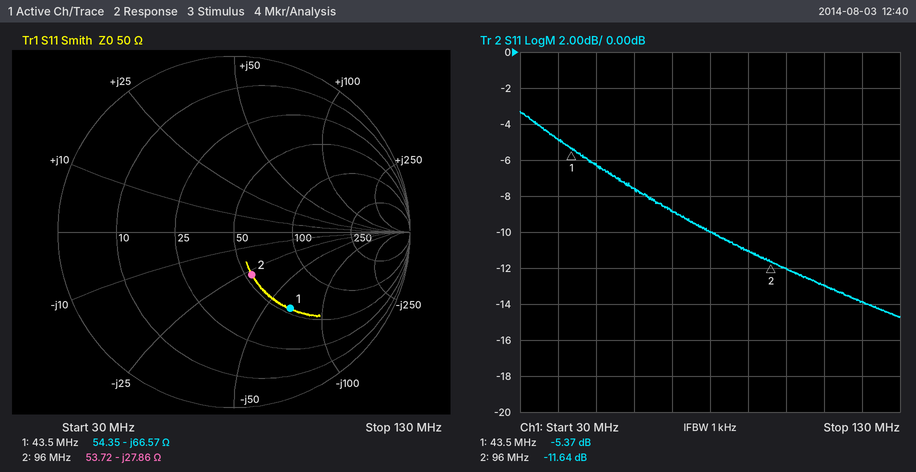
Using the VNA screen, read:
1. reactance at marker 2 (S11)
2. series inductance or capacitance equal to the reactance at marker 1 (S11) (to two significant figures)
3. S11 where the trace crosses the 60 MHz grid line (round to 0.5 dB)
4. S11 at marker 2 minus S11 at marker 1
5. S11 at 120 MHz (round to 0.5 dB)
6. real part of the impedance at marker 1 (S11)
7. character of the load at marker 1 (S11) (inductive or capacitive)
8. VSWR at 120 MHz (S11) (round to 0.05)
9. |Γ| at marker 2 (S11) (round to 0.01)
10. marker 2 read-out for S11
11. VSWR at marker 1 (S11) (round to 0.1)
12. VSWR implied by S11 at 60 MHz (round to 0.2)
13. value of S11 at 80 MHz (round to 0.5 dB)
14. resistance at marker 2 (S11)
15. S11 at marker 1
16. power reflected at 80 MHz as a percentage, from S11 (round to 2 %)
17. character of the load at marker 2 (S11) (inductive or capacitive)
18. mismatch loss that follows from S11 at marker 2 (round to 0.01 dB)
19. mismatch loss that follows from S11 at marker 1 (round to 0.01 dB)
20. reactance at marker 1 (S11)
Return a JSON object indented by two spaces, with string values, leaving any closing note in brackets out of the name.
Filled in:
{
  "reactance at marker 2": "-27.86 Ω",
  "series inductance or capacitance equal to the reactance at marker 1 (S11)": "55 pF",
  "S11 where the trace crosses the 60 MHz grid line": "-7.5 dB",
  "S11 at marker 2 minus S11 at marker 1": "-6.27 dB",
  "S11 at 120 MHz": "-14.0 dB",
  "real part of the impedance at marker 1": "54.35 Ω",
  "character of the load at marker 1 (S11)": "capacitive",
  "VSWR at 120 MHz (S11)": "1.50",
  "|Γ| at marker 2 (S11)": "0.26",
  "marker 2 read-out for S11": "-11.64 dB",
  "VSWR at marker 1 (S11)": "3.3",
  "VSWR implied by S11 at 60 MHz": "2.4",
  "value of S11 at 80 MHz": "-10.0 dB",
  "resistance at marker 2": "53.72 Ω",
  "S11 at marker 1": "-5.37 dB",
  "power reflected at 80 MHz as a percentage, from S11": "10 %",
  "character of the load at marker 2 (S11)": "capacitive",
  "mismatch loss that follows from S11 at marker 2": "0.31 dB",
  "mismatch loss that follows from S11 at marker 1": "1.49 dB",
  "reactance at marker 1": "-66.57 Ω"
}
